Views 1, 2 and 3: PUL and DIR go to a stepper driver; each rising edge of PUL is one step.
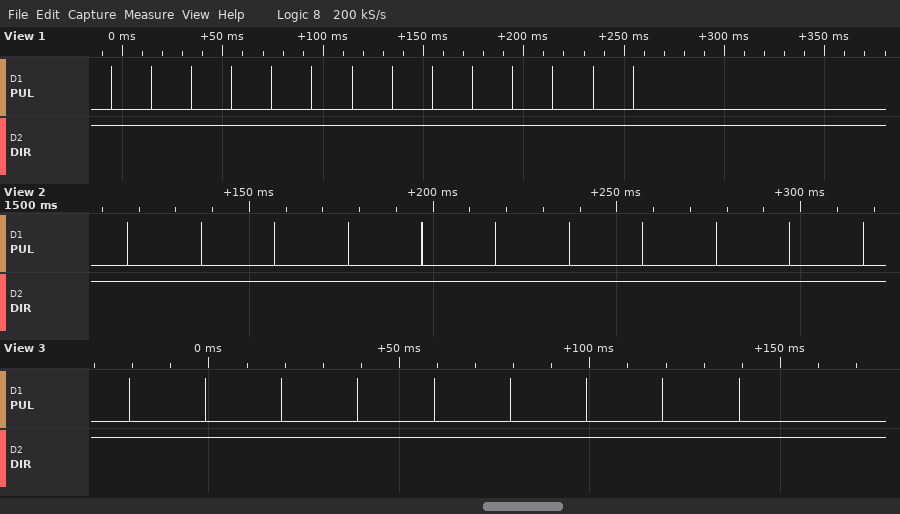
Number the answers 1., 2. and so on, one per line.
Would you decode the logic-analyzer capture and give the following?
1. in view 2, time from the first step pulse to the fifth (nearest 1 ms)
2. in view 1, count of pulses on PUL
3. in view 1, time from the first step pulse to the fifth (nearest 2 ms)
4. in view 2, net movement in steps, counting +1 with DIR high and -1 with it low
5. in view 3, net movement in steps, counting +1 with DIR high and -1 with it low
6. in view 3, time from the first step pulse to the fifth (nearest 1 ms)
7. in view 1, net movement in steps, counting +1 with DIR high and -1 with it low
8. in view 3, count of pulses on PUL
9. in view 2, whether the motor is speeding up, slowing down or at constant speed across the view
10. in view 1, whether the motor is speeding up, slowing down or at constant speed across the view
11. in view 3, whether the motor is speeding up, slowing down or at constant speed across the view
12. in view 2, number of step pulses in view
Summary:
1. 80 ms
2. 14
3. 80 ms
4. +11
5. +9
6. 80 ms
7. +14
8. 9
9. constant speed
10. constant speed
11. constant speed
12. 11
